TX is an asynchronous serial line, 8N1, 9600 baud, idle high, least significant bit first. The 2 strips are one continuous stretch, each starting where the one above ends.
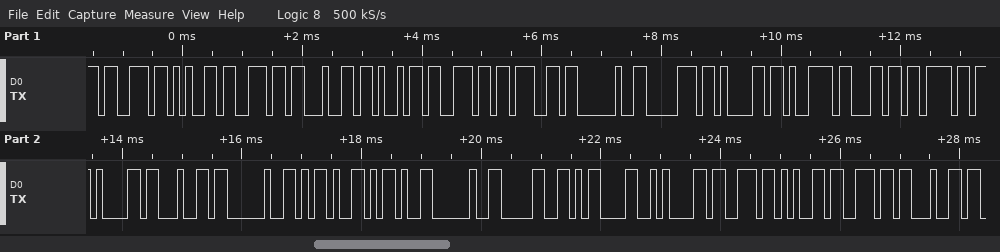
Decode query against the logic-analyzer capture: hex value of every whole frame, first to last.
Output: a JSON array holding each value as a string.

["0x73 0x65 0x6E 0x64 0x69 0x6E 0x67 0x20 0x70 0x61 0x79 0x6C 0x6F 0x61 0x64 0x20 0x2D 0x2D 0x20 0x30 0x0D 0x0A 0x73 0x65 0x6E 0x64"]
